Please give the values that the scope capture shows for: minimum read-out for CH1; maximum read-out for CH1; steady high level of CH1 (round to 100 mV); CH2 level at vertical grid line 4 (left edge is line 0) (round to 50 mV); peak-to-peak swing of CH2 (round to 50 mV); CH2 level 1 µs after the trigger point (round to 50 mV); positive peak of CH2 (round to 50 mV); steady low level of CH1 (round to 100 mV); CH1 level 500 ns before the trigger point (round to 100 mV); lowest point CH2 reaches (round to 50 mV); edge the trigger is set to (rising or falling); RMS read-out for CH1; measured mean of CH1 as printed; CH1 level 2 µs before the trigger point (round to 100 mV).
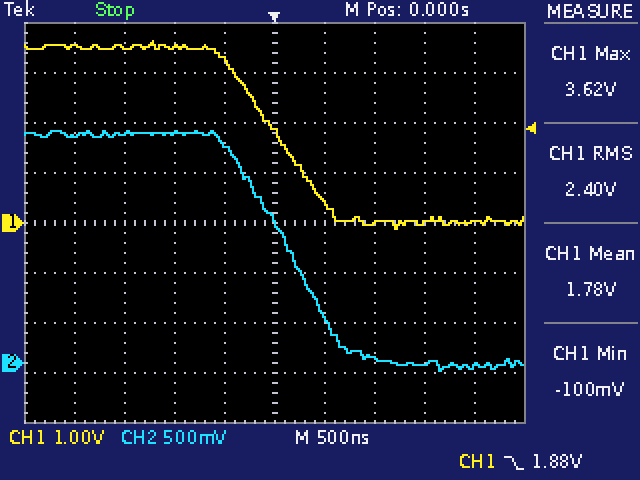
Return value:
-100 mV
3.62 V
3.5 V
2.20 V
2.40 V
50 mV
2.30 V
0.0 V
3.2 V
-100 mV
falling
2.40 V
1.78 V
3.5 V
